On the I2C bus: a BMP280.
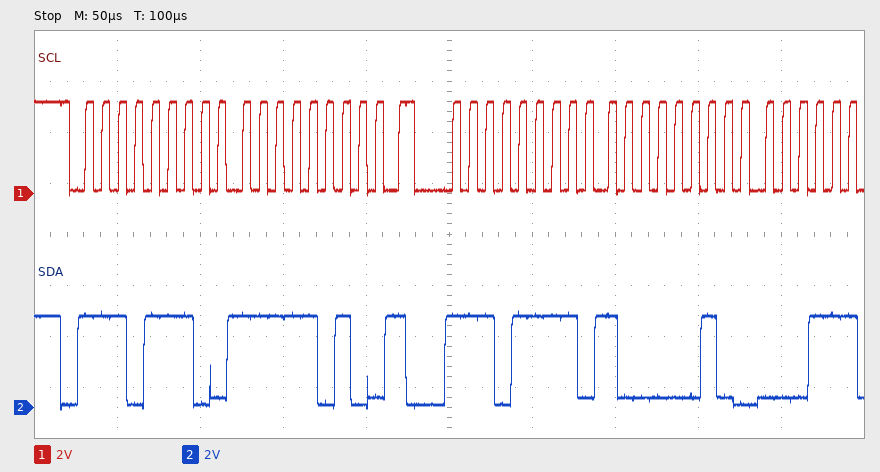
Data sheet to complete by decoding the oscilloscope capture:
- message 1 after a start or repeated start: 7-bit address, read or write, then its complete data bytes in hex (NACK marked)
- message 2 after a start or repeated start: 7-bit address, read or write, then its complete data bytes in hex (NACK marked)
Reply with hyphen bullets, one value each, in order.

- 0x77 write: FA
- 0x77 read: 82
